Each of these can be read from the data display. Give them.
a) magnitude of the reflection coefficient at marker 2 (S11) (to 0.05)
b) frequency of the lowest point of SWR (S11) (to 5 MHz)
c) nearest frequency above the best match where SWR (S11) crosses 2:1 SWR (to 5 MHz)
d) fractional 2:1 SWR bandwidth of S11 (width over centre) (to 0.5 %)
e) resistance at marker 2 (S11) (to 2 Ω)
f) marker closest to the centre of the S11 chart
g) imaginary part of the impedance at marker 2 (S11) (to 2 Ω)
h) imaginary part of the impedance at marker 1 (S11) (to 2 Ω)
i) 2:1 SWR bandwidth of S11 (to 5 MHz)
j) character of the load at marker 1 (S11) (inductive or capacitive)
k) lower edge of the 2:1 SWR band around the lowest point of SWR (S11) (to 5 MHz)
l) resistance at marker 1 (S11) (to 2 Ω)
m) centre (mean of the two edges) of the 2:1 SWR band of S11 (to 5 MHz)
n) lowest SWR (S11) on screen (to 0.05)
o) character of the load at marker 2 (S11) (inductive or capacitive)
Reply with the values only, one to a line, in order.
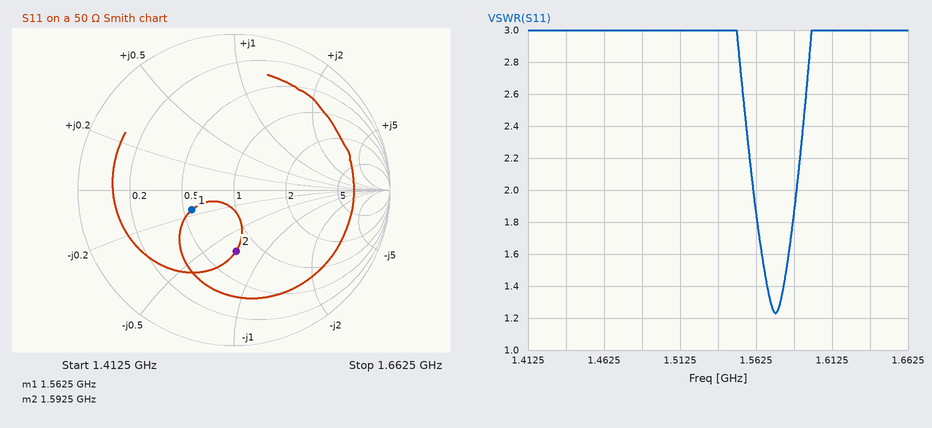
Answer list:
0.40
1.575 GHz
1.590 GHz
2.0 %
38 Ω
marker 1
-34 Ω
-8 Ω
30 MHz
capacitive
1.560 GHz
28 Ω
1.575 GHz
1.25
capacitive
